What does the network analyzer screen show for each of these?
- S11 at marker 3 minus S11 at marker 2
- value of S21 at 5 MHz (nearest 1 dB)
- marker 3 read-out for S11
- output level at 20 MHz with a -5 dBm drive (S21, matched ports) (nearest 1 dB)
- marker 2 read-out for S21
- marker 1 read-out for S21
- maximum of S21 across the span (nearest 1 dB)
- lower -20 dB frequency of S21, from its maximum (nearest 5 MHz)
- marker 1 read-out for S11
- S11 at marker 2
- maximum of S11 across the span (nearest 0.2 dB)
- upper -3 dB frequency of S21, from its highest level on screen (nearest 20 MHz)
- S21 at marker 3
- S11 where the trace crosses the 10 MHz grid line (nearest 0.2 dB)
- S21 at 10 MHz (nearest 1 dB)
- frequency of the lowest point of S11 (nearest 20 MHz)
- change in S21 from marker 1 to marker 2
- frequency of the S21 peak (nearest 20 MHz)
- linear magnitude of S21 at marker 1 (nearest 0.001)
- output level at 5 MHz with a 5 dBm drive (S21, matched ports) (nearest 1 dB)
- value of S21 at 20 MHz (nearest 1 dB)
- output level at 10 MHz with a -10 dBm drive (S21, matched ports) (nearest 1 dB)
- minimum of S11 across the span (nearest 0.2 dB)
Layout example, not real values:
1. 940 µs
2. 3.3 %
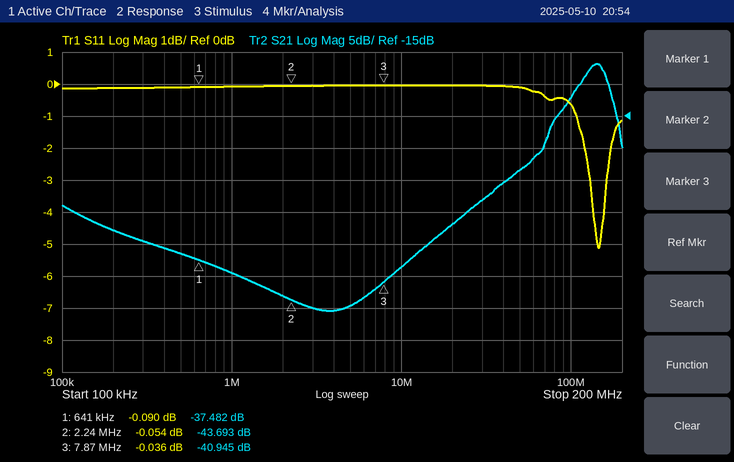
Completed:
1. 0.018 dB
2. -45 dB
3. -0.036 dB
4. -37 dBm
5. -43.693 dB
6. -37.482 dB
7. -7 dB
8. 35 MHz
9. -0.090 dB
10. -0.054 dB
11. 0.0 dB
12. 160 MHz
13. -40.945 dB
14. 0.0 dB
15. -39 dB
16. 140 MHz
17. -6.211 dB
18. 140 MHz
19. 0.013
20. -40 dBm
21. -32 dB
22. -49 dBm
23. -5.2 dB
